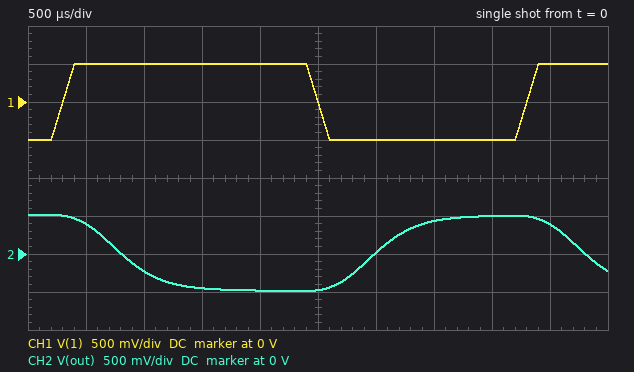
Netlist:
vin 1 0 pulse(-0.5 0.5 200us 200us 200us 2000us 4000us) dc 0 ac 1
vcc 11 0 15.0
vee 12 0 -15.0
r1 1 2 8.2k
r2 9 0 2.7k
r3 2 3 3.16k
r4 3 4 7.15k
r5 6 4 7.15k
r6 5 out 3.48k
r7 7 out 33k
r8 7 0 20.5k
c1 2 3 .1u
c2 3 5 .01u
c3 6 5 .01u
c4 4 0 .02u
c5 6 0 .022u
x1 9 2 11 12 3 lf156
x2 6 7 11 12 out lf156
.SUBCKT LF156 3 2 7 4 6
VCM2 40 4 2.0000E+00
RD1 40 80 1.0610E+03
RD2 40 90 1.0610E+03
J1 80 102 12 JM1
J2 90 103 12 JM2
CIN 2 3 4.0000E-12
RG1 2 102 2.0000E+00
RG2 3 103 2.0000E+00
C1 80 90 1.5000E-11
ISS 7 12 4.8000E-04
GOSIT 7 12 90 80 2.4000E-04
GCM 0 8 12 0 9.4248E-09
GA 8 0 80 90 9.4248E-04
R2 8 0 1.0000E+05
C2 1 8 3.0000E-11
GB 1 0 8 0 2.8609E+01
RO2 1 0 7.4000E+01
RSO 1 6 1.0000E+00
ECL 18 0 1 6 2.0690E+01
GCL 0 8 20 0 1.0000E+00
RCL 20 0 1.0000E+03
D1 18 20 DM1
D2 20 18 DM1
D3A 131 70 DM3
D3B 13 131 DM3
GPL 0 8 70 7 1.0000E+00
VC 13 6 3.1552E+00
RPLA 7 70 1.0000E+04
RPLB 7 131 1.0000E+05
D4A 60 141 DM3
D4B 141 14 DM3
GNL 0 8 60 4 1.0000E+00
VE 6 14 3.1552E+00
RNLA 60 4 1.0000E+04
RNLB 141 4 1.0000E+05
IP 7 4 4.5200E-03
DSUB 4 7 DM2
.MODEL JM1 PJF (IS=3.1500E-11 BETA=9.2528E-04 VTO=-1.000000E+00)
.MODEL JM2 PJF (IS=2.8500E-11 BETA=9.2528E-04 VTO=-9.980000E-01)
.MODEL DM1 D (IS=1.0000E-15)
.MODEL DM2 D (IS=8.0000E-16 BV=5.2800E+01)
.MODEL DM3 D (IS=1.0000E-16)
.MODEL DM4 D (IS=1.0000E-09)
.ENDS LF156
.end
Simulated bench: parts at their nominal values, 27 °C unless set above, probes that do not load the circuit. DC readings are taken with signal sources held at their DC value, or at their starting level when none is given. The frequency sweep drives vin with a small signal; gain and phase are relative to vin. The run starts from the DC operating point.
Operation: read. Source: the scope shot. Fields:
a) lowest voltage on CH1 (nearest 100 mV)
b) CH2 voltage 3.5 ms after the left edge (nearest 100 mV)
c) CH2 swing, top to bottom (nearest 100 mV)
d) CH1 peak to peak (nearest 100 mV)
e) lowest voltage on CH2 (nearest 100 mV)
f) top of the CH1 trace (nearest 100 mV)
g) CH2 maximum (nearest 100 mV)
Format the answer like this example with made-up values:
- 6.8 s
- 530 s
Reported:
- -500 mV
- 400 mV
- 1.0 V
- 1.0 V
- -500 mV
- 500 mV
- 500 mV
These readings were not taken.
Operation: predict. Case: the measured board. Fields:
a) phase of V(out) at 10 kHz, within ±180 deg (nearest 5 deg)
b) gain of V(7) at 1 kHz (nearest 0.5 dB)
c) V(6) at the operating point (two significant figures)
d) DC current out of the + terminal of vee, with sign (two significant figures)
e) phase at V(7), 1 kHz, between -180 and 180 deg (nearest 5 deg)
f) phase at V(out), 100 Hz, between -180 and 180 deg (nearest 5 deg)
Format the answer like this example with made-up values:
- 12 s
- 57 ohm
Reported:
- 100 deg
- -20.0 dB
- 2.8 mV
- -10 mA
- 25 deg
- 160 deg
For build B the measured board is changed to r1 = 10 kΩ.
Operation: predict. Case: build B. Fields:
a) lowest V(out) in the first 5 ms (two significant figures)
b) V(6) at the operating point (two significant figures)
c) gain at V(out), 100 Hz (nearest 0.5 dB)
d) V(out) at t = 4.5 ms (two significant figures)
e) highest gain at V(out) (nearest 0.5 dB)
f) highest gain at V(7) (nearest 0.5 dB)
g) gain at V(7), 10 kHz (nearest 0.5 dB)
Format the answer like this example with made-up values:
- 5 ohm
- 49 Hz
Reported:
- -400 mV
- 2.6 mV
- -2.0 dB
- 320 mV
- -1.5 dB
- -10.0 dB
- -51.0 dB
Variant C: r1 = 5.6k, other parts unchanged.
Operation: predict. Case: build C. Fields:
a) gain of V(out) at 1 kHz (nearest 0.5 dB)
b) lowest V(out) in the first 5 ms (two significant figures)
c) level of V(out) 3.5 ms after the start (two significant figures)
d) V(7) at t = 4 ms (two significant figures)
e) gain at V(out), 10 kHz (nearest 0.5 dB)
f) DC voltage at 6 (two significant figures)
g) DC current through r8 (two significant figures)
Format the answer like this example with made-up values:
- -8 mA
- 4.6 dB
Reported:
- -8.5 dB
- -720 mV
- 630 mV
- 280 mV
- -37.5 dB
- 3.1 mV
- 250 nA
